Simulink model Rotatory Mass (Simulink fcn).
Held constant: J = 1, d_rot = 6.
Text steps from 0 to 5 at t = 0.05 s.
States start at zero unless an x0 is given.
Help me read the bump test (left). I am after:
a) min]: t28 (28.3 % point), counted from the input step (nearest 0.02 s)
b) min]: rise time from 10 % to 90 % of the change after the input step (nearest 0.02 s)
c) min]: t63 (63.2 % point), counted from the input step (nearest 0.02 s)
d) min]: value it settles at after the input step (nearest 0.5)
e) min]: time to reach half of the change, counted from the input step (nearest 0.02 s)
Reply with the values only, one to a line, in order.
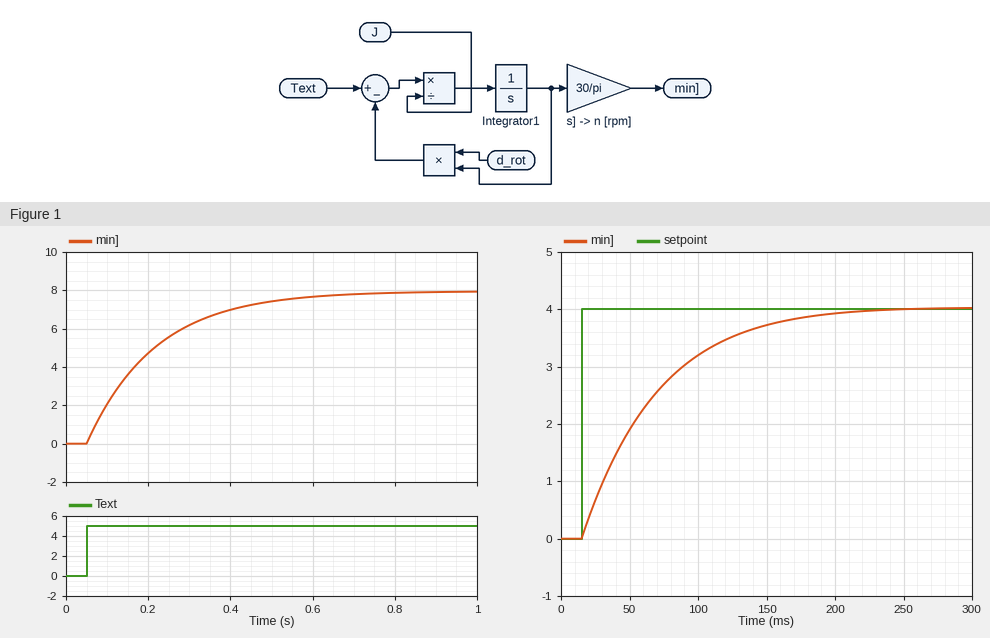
0.06 s
0.36 s
0.16 s
8.0
0.12 s
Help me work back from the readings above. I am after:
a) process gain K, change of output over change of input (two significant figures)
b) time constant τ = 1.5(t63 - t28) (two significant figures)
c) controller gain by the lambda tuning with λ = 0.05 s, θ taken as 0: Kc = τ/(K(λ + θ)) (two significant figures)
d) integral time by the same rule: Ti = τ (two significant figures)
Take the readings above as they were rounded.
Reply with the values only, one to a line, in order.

1.6
0.15 s
1.9
0.15 s
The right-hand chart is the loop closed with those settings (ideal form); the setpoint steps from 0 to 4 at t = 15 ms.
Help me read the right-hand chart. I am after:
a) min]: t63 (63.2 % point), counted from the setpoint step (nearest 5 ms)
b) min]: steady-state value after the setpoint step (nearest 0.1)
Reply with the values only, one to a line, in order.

55 ms
4.0
